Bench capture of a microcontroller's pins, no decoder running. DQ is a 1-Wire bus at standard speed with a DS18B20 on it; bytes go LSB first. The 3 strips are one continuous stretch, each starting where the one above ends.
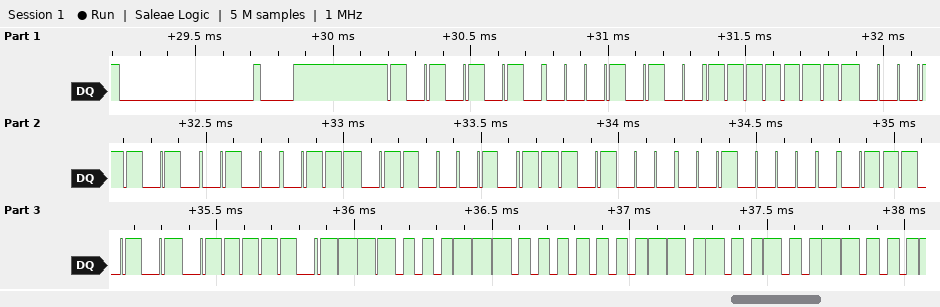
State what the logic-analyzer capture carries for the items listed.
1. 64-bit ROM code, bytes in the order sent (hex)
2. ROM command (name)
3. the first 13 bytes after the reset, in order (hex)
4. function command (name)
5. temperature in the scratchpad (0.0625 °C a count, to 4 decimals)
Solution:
28 FF 58 E2 46 17 04 AE
Match ROM
55 28 FF 58 E2 46 17 04 AE BE C7 01 4B
Read Scratchpad
28.4375 °C
